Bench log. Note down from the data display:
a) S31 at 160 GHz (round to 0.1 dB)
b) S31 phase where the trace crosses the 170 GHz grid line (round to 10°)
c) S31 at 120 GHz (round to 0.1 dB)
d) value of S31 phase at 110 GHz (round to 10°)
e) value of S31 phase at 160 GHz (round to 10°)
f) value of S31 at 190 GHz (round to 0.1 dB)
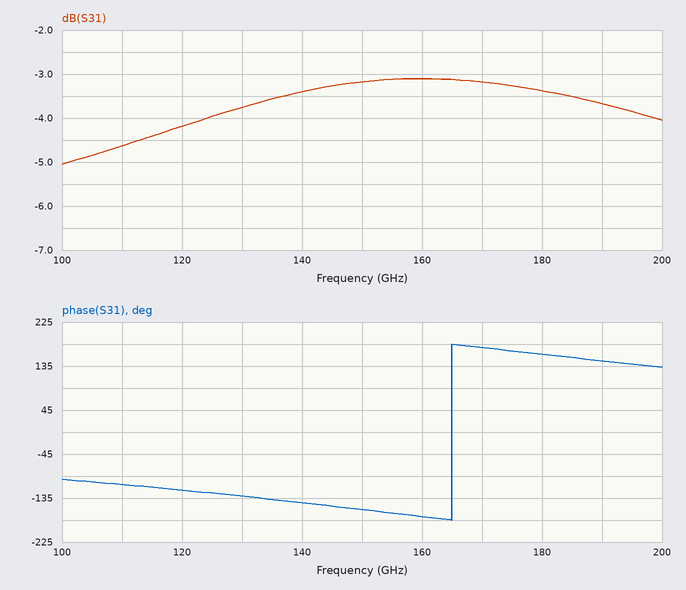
-3.1 dB
170°
-4.2 dB
-110°
-170°
-3.7 dB
